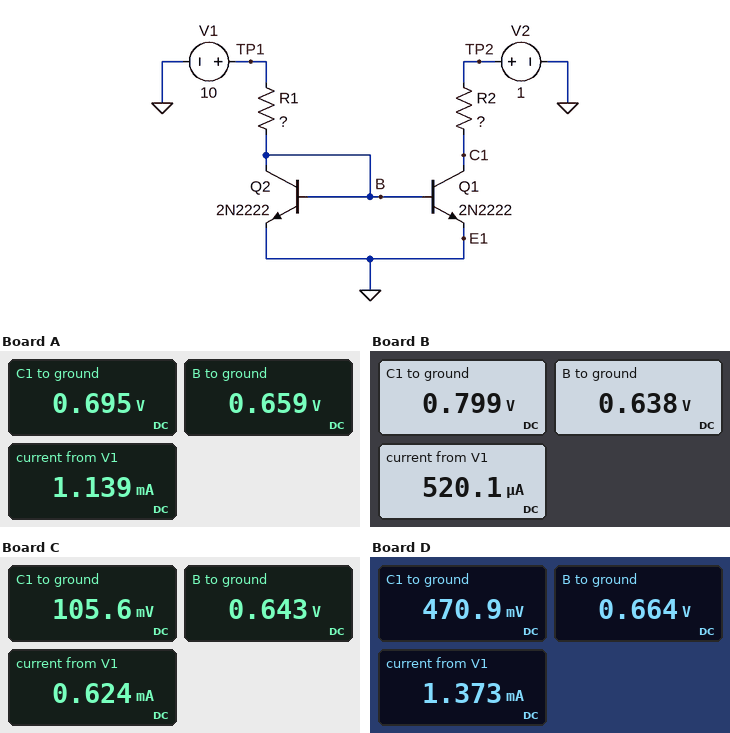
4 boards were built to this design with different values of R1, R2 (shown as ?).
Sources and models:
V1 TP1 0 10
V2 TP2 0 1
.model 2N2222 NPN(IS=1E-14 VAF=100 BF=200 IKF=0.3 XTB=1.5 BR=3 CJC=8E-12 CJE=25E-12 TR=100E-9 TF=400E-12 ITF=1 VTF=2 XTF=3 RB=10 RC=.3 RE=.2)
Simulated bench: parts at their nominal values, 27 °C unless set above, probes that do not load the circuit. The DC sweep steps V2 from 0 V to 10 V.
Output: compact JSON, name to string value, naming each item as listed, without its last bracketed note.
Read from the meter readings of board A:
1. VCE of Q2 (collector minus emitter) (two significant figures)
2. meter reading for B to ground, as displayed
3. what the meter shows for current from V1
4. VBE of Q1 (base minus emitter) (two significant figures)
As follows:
{"VCE of Q2 (collector minus emitter)": "660 mV", "meter reading for B to ground, as displayed": "0.659 V", "what the meter shows for current from V1": "1.139 mA", "VBE of Q1 (base minus emitter)": "660 mV"}
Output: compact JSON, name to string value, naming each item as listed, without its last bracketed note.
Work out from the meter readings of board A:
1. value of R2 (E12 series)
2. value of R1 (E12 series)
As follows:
{"value of R2": "270 Ω", "value of R1": "8.2 kΩ"}
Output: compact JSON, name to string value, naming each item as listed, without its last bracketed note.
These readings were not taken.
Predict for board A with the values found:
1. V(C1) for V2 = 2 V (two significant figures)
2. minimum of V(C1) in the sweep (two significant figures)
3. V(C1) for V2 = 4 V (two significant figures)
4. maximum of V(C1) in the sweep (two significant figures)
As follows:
{"V(C1) for V2 = 2 V": "1.7 V", "minimum of V(C1) in the sweep": "6.8 mV", "V(C1) for V2 = 4 V": "3.7 V", "maximum of V(C1) in the sweep": "9.7 V"}
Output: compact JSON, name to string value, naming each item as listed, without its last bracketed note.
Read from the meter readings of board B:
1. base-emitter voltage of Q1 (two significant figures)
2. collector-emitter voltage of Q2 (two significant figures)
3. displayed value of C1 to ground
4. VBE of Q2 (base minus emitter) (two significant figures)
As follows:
{"base-emitter voltage of Q1": "640 mV", "collector-emitter voltage of Q2": "640 mV", "displayed value of C1 to ground": "0.799 V", "VBE of Q2 (base minus emitter)": "640 mV"}
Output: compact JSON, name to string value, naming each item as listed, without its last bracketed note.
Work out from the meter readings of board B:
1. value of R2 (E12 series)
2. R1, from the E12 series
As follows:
{"value of R2": "390 Ω", "R1, from the E12 series": "18 kΩ"}
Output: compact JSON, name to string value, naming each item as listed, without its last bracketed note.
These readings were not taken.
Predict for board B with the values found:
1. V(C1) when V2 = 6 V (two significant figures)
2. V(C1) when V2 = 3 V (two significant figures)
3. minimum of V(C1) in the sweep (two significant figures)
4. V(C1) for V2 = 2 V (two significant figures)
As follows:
{"V(C1) when V2 = 6 V": "5.8 V", "V(C1) when V2 = 3 V": "2.8 V", "minimum of V(C1) in the sweep": "6.4 mV", "V(C1) for V2 = 2 V": "1.8 V"}
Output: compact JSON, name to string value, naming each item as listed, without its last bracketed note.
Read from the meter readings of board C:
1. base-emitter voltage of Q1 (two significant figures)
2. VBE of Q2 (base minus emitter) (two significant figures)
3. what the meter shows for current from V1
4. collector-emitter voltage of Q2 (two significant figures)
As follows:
{"base-emitter voltage of Q1": "640 mV", "VBE of Q2 (base minus emitter)": "640 mV", "what the meter shows for current from V1": "0.624 mA", "collector-emitter voltage of Q2": "640 mV"}
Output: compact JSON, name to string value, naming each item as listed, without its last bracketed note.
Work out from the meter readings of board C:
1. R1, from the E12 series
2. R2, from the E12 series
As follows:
{"R1, from the E12 series": "15 kΩ", "R2, from the E12 series": "1.5 kΩ"}
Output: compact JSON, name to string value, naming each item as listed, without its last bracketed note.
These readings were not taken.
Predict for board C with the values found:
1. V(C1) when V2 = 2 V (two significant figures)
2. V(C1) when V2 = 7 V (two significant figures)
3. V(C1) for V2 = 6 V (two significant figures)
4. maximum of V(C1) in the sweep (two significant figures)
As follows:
{"V(C1) when V2 = 2 V": "1.1 V", "V(C1) when V2 = 7 V": "6.0 V", "V(C1) for V2 = 6 V": "5.0 V", "maximum of V(C1) in the sweep": "9.0 V"}
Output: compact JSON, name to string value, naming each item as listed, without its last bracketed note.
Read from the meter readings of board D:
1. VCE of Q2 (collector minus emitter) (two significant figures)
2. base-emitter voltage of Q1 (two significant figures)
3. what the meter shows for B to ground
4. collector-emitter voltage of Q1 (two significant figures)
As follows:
{"VCE of Q2 (collector minus emitter)": "660 mV", "base-emitter voltage of Q1": "660 mV", "what the meter shows for B to ground": "0.664 V", "collector-emitter voltage of Q1": "470 mV"}
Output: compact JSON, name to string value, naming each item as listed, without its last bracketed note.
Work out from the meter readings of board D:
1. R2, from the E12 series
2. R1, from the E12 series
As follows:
{"R2, from the E12 series": "390 Ω", "R1, from the E12 series": "6.8 kΩ"}
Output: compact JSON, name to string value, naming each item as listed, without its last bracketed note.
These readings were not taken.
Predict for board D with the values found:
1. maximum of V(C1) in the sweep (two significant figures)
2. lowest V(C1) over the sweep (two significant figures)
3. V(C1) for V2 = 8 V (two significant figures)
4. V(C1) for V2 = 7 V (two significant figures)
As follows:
{"maximum of V(C1) in the sweep": "9.4 V", "lowest V(C1) over the sweep": "7.1 mV", "V(C1) for V2 = 8 V": "7.4 V", "V(C1) for V2 = 7 V": "6.4 V"}
